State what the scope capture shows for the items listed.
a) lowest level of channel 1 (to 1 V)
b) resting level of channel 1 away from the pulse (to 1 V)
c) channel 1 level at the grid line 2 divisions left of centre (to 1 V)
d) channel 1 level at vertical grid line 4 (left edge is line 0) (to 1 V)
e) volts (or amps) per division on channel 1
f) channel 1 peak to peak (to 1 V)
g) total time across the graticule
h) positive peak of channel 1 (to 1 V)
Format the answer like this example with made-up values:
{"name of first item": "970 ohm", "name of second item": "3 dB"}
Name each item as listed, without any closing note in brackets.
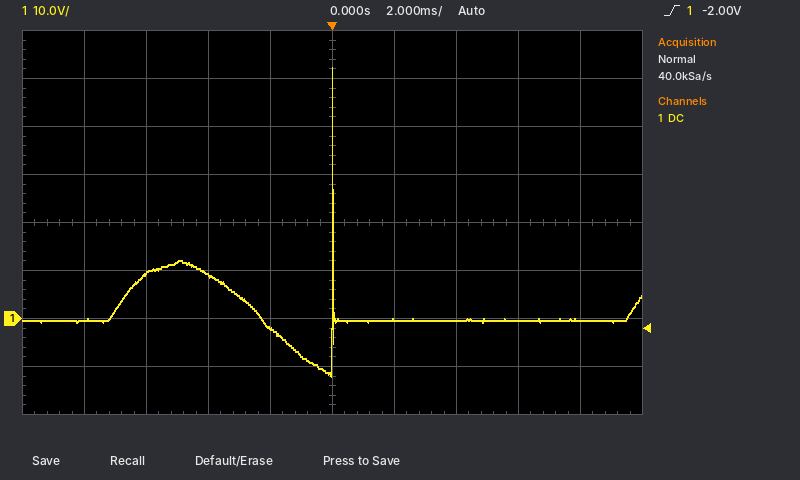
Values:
{"lowest level of channel 1": "-12 V", "resting level of channel 1 away from the pulse": "0 V", "channel 1 level at the grid line 2 divisions left of centre": "9 V", "channel 1 level at vertical grid line 4 (left edge is line 0)": "-2 V", "volts (or amps) per division on channel 1": "10 V", "channel 1 peak to peak": "64 V", "total time across the graticule": "20 ms", "positive peak of channel 1": "52 V"}
